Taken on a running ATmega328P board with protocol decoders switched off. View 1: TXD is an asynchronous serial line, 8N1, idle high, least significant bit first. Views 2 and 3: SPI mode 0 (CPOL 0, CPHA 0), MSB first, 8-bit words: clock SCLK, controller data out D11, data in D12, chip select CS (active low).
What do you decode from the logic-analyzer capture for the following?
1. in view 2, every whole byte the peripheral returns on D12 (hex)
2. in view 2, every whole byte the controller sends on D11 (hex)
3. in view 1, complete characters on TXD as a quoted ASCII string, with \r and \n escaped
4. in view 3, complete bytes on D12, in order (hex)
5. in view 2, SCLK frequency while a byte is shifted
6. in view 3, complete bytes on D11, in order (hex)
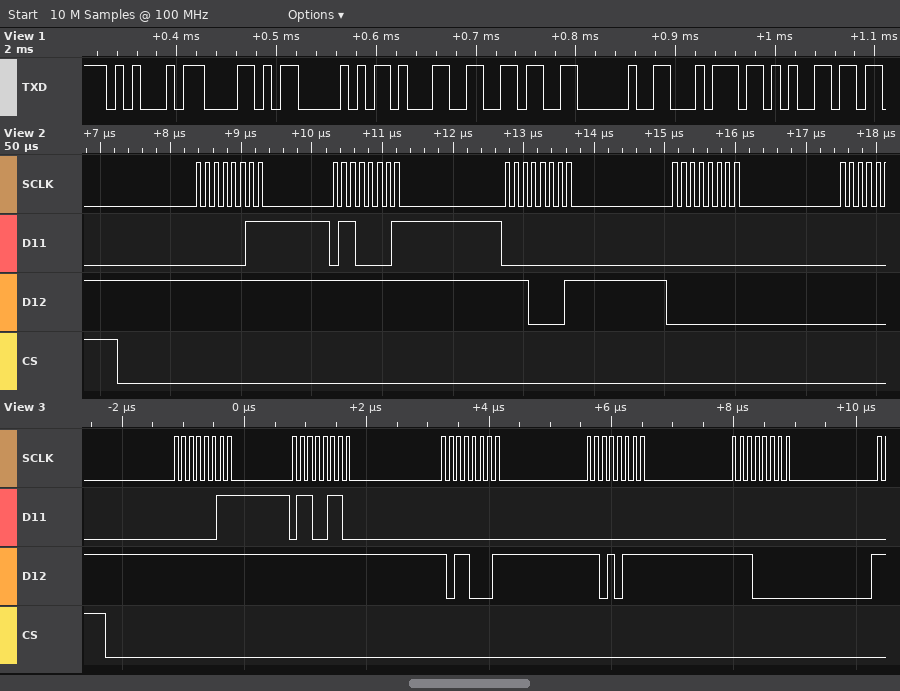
0xFF 0xFF 0xE1 0x00
0x03 0x61 0x00 0x00
"EXP16 te"
0xFF 0xFF 0xB1 0xD7 0xE0
8 MHz
0x03 0x66 0x00 0x00 0x00
